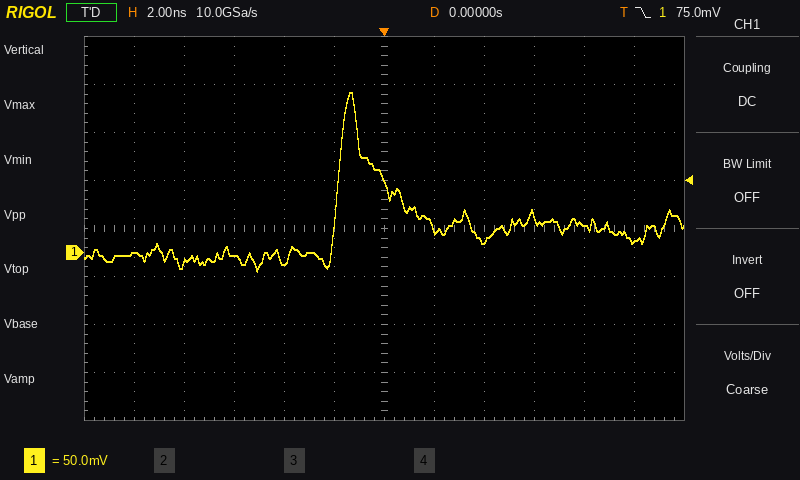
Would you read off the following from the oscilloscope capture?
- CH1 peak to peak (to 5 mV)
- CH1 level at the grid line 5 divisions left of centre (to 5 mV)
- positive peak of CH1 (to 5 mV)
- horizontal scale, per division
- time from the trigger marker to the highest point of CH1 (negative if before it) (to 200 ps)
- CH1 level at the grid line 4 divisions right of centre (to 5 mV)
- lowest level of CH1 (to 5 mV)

185 mV
0 mV
165 mV
2 ns
-1.4 ns
30 mV
-20 mV
